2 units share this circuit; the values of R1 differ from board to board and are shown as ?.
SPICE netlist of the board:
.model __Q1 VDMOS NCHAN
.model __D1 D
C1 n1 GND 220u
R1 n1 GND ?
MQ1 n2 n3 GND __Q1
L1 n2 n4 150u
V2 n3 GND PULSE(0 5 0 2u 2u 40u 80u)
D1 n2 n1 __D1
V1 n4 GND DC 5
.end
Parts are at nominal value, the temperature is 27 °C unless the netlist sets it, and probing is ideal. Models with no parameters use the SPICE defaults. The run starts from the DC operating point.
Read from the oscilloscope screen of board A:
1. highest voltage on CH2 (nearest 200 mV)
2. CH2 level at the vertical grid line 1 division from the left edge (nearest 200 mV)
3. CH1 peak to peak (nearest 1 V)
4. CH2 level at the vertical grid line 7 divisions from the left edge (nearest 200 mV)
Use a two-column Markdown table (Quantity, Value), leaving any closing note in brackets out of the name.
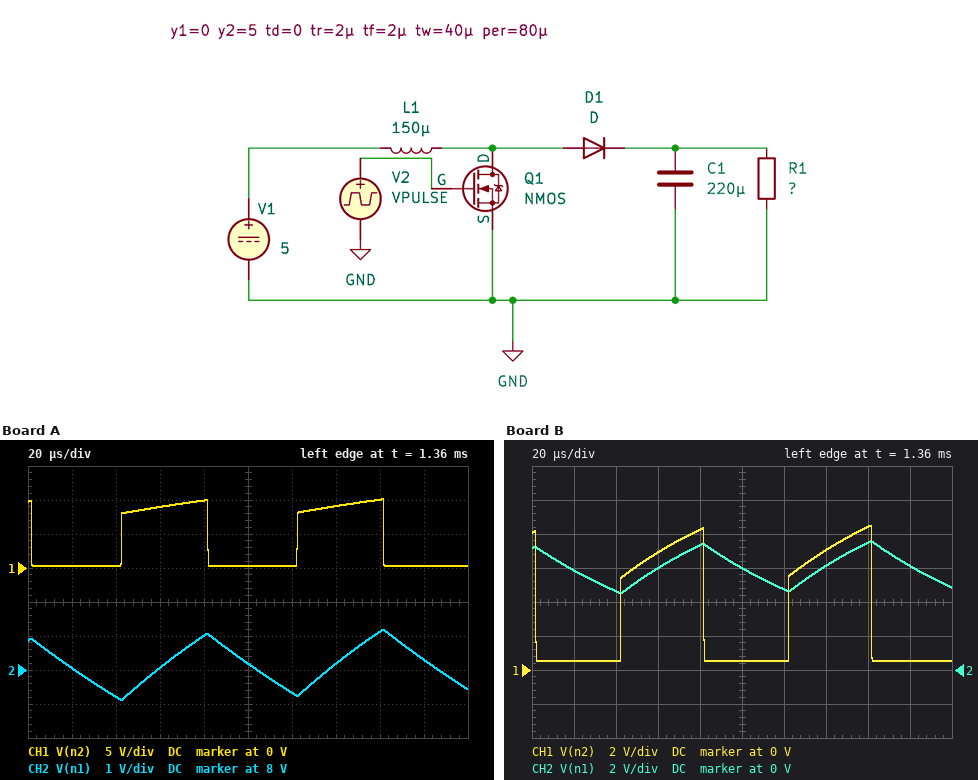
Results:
| Quantity | Value |
|---|---|
| highest voltage on CH2 | 9.2 V |
| CH2 level at the vertical grid line 1 division from the left edge | 8.0 V |
| CH1 peak to peak | 10 V |
| CH2 level at the vertical grid line 7 divisions from the left edge | 8.2 V |
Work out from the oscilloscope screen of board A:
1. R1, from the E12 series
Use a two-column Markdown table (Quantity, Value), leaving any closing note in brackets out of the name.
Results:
| Quantity | Value |
|---|---|
| R1, from the E12 series | 0.82 Ω |
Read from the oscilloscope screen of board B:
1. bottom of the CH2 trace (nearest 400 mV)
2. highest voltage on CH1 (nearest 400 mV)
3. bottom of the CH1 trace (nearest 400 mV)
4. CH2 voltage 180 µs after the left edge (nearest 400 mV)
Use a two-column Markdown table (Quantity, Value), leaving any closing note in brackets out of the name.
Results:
| Quantity | Value |
|---|---|
| bottom of the CH2 trace | 4.4 V |
| highest voltage on CH1 | 8.4 V |
| bottom of the CH1 trace | 400 mV |
| CH2 voltage 180 µs after the left edge | 6.0 V |
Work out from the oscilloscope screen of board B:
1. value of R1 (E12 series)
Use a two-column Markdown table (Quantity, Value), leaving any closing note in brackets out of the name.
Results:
| Quantity | Value |
|---|---|
| value of R1 | 0.39 Ω |
